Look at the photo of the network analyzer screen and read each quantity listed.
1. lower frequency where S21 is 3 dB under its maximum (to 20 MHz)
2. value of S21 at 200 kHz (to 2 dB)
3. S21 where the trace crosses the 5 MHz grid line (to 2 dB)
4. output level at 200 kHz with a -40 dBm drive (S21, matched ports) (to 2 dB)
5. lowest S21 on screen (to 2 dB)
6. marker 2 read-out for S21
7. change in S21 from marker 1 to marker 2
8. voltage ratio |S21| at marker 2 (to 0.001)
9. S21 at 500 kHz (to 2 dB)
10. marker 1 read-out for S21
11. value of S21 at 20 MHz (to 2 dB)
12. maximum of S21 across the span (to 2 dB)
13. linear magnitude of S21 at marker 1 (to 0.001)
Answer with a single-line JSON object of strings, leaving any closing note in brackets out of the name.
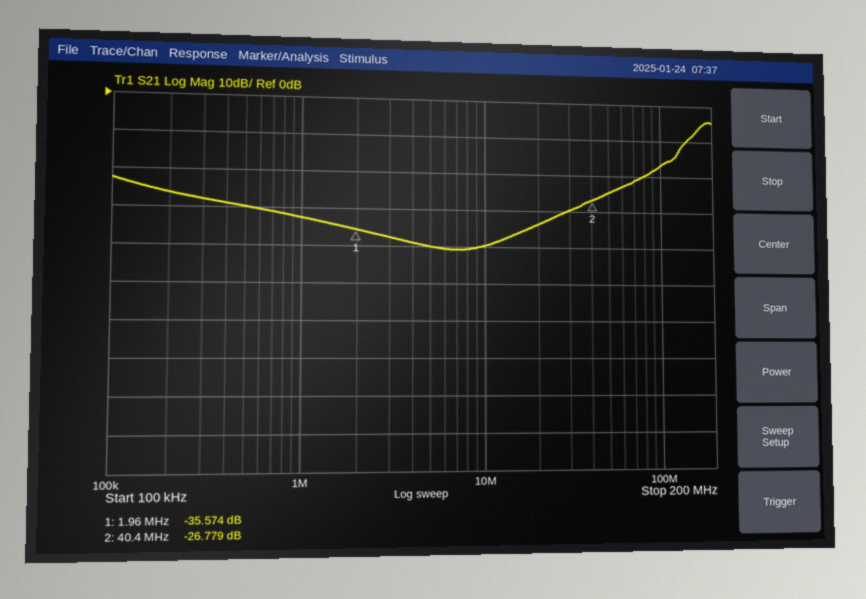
{"lower frequency where S21 is 3 dB under its maximum": "160 MHz", "value of S21 at 200 kHz": "-26 dB", "S21 where the trace crosses the 5 MHz grid line": "-40 dB", "output level at 200 kHz with a -40 dBm drive (S21, matched ports)": "-66 dBm", "lowest S21 on screen": "-40 dB", "marker 2 read-out for S21": "-26.779 dB", "change in S21 from marker 1 to marker 2": "8.795 dB", "voltage ratio |S21| at marker 2": "0.046", "S21 at 500 kHz": "-30 dB", "marker 1 read-out for S21": "-35.574 dB", "value of S21 at 20 MHz": "-34 dB", "maximum of S21 across the span": "-4 dB", "linear magnitude of S21 at marker 1": "0.017"}
